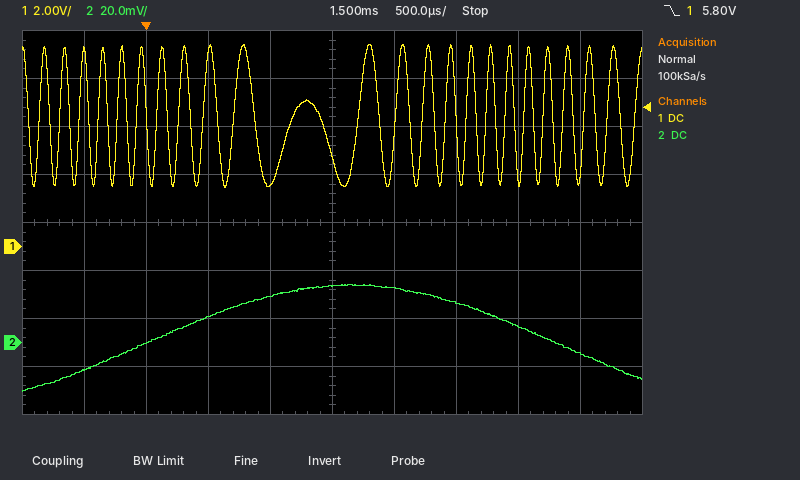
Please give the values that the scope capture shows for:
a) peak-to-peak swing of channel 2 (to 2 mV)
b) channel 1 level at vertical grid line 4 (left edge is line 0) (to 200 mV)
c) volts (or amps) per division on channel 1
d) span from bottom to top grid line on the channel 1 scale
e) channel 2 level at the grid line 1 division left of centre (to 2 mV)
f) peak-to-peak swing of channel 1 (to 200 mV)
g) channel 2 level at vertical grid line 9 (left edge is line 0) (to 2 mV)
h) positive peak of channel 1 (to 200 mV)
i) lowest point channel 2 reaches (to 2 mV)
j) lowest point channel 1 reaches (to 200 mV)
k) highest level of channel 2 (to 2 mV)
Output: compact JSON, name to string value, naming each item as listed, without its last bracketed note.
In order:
{"peak-to-peak swing of channel 2": "44 mV", "channel 1 level at vertical grid line 4 (left edge is line 0)": "2.6 V", "volts (or amps) per division on channel 1": "2 V", "span from bottom to top grid line on the channel 1 scale": "16 V", "channel 2 level at the grid line 1 division left of centre": "20 mV", "peak-to-peak swing of channel 1": "6.0 V", "channel 2 level at vertical grid line 9 (left edge is line 0)": "-4 mV", "positive peak of channel 1": "8.4 V", "lowest point channel 2 reaches": "-20 mV", "lowest point channel 1 reaches": "2.4 V", "highest level of channel 2": "24 mV"}
